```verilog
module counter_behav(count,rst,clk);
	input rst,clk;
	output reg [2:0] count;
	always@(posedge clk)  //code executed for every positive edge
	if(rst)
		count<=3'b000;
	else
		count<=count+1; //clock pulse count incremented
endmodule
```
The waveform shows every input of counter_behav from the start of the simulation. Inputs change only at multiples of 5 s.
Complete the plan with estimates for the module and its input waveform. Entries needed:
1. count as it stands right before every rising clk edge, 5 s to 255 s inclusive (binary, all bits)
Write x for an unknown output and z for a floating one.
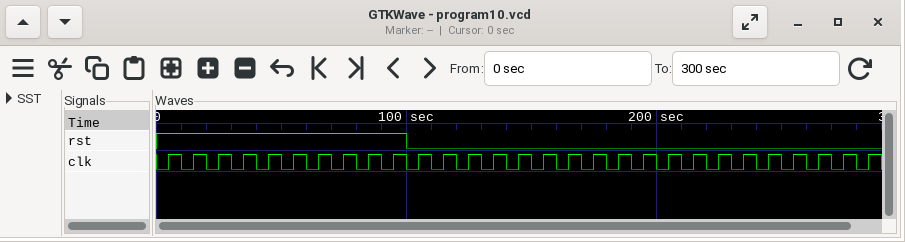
x, 000, 000, 000, 000, 000, 000, 000, 000, 000, 000, 001, 010, 011, 100, 101, 110, 111, 000, 001, 010, 011, 100, 101, 110, 111
